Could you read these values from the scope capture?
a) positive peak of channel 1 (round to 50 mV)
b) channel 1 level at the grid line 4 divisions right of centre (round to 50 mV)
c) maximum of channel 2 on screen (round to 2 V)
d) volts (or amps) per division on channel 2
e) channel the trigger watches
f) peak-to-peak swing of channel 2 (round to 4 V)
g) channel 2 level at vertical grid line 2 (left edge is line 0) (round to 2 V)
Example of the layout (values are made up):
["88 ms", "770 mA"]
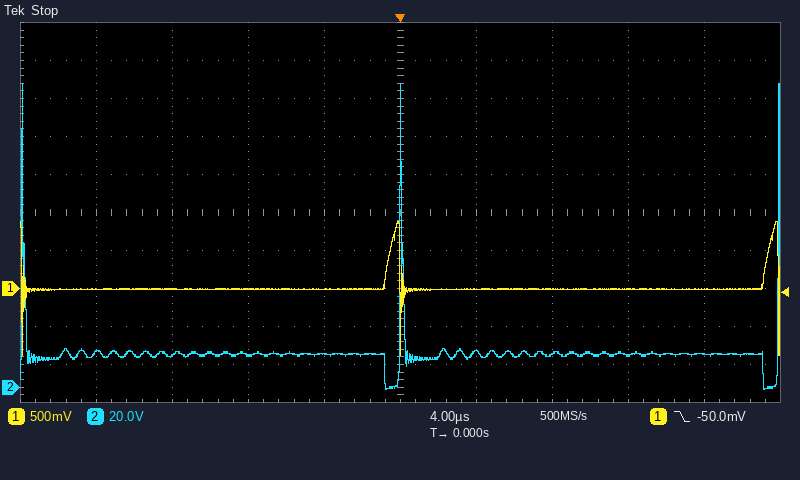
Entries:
["900 mV", "0 mV", "160 V", "20 V", "channel 1", "160 V", "18 V"]
